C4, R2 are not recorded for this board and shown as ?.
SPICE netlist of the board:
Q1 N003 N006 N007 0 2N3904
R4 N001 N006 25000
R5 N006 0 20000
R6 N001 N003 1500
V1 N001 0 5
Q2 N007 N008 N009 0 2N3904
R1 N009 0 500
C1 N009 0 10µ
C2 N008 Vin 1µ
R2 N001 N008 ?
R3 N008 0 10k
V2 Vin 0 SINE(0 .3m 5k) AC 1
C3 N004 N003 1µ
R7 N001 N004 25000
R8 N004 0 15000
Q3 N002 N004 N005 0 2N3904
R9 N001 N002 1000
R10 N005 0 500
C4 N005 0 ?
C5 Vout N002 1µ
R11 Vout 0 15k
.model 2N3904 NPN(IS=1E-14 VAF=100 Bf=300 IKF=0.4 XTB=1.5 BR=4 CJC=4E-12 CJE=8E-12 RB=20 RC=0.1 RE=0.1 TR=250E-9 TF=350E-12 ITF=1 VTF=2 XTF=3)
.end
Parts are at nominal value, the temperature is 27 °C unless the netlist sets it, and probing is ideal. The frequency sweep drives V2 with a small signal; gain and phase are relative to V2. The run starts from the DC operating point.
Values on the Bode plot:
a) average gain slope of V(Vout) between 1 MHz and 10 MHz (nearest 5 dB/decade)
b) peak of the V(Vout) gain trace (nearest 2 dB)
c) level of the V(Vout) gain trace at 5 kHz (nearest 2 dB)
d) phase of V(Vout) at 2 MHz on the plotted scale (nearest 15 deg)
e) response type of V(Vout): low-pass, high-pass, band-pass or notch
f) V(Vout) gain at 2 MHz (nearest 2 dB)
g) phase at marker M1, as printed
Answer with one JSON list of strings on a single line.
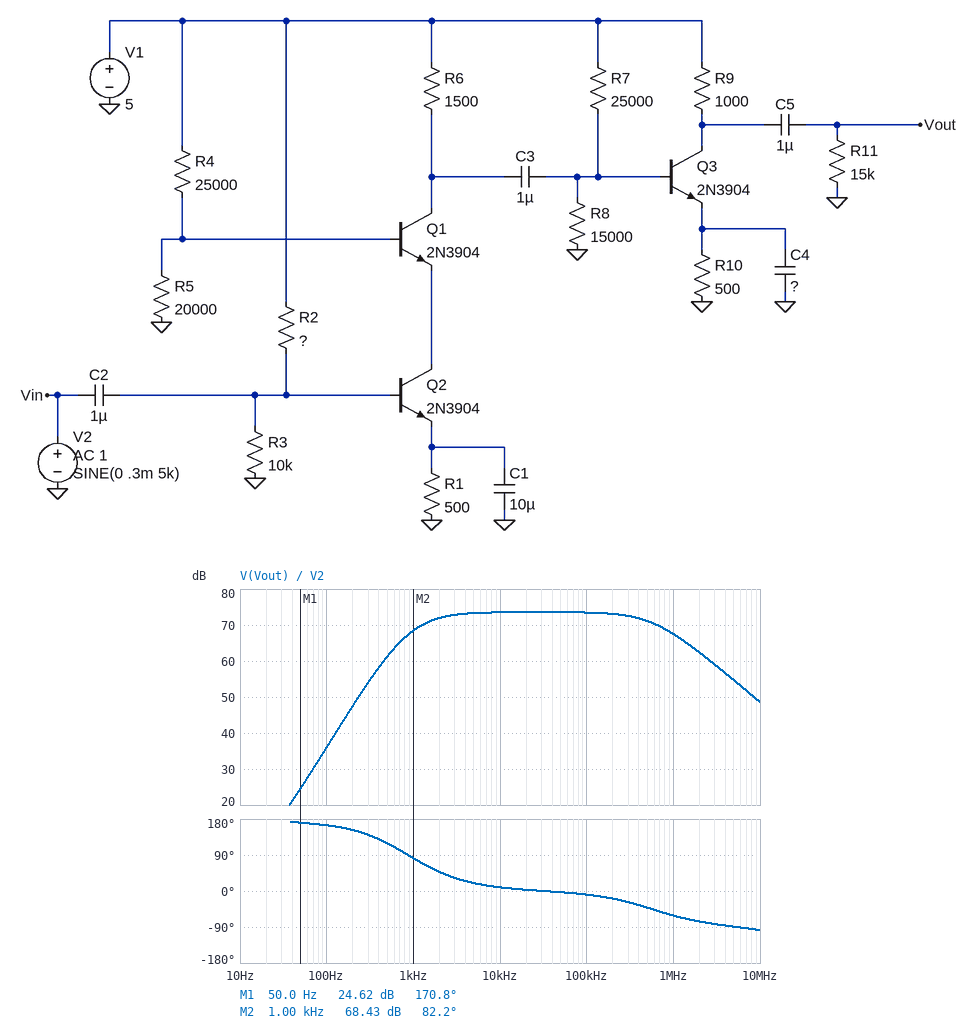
["-20 dB/decade", "74 dB", "74 dB", "-75 deg", "band-pass", "62 dB", "170.8 deg"]
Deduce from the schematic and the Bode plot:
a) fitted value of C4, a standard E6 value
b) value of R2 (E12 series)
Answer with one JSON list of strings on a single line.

["15 µF", "22 kΩ"]
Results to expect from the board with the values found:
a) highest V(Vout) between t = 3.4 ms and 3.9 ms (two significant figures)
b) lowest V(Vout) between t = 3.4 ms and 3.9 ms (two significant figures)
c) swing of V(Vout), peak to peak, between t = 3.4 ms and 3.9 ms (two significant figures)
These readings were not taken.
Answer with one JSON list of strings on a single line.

["1.2 V", "-1.4 V", "2.6 V"]
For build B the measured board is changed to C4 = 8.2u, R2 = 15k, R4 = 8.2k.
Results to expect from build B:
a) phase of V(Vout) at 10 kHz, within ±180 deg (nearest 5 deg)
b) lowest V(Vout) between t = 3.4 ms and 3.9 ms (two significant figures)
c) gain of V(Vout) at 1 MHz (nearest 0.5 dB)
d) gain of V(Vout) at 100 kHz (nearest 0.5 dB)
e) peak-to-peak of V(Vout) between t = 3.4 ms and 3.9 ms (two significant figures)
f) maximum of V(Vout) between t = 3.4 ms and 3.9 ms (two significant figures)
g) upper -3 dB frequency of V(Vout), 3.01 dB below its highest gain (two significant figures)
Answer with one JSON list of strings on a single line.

["15 deg", "-1.5 V", "70.0 dB", "75.5 dB", "2.8 V", "1.3 V", "640 kHz"]
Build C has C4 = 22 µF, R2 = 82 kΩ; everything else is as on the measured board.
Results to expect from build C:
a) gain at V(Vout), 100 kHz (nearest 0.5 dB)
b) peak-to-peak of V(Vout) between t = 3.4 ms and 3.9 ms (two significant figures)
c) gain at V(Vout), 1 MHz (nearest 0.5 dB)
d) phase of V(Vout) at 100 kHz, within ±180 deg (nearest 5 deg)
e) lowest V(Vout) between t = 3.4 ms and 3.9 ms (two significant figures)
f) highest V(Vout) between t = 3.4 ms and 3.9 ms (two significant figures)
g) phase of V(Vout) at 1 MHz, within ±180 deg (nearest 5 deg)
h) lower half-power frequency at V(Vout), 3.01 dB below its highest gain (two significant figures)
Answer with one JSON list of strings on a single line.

["29.5 dB", "18 mV", "23.5 dB", "-10 deg", "-9.2 mV", "9.2 mV", "-75 deg", "480 Hz"]
